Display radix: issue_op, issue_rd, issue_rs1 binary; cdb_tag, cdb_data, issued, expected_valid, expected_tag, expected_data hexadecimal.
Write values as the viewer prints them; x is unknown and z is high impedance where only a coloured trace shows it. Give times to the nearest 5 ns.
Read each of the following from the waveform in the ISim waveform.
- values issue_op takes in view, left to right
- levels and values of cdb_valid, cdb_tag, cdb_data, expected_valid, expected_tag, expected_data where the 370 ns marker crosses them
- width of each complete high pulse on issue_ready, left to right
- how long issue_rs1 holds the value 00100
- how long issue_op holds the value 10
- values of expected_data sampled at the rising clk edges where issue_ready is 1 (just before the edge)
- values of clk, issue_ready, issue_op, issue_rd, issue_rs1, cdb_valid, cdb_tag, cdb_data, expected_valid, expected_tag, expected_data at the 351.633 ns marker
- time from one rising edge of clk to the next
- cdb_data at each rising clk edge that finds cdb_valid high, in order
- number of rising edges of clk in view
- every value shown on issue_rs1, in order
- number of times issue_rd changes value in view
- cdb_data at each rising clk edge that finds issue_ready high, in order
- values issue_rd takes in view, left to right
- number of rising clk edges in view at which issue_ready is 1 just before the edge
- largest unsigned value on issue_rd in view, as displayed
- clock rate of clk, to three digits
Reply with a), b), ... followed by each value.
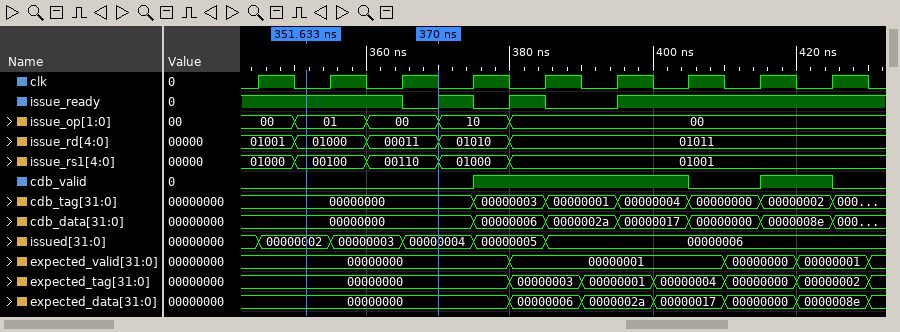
a) 00, 01, 00, 10, 00
b) cdb_valid=0, cdb_tag=00000000, cdb_data=00000000, expected_valid=00000000, expected_tag=00000000, expected_data=00000000
c) 5 ns, 5 ns
d) 10 ns
e) 10 ns
f) 00000000, 00000000, 00000000, 00000000, 00000006, 00000017, 00000000, 0000008e
g) clk=0, issue_ready=1, issue_op=01, issue_rd=01000, issue_rs1=00100, cdb_valid=0, cdb_tag=00000000, cdb_data=00000000, expected_valid=00000000, expected_tag=00000000, expected_data=00000000
h) 10 ns
i) 00000006, 0000002a, 00000017, 0000008e
j) 9
k) 01000, 00100, 00110, 01000, 01001
l) 4
m) 00000000, 00000000, 00000000, 00000000, 00000006, 00000017, 00000000, 0000008e
n) 01001, 01000, 00011, 01010, 01011
o) 8
p) 01011
q) 100 MHz
